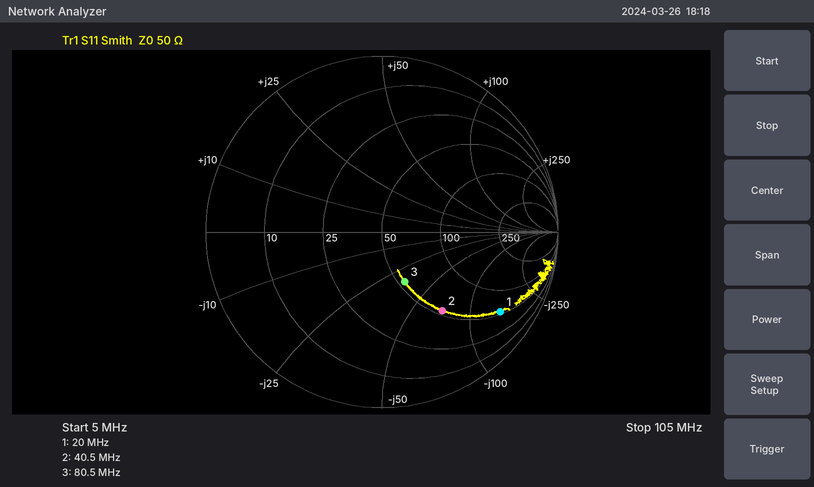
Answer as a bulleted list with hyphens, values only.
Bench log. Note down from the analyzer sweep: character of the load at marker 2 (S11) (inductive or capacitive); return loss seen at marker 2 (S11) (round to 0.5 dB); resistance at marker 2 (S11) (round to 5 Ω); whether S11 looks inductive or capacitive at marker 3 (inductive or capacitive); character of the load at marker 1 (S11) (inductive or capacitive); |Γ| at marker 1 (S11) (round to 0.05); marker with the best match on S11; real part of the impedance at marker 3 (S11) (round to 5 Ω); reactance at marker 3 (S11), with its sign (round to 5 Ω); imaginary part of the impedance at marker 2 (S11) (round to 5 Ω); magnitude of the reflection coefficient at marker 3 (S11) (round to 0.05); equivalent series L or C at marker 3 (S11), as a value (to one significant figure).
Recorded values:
- capacitive
- 5.0 dB
- 55 Ω
- capacitive
- capacitive
- 0.80
- marker 3
- 55 Ω
- -35 Ω
- -70 Ω
- 0.30
- 60 pF
